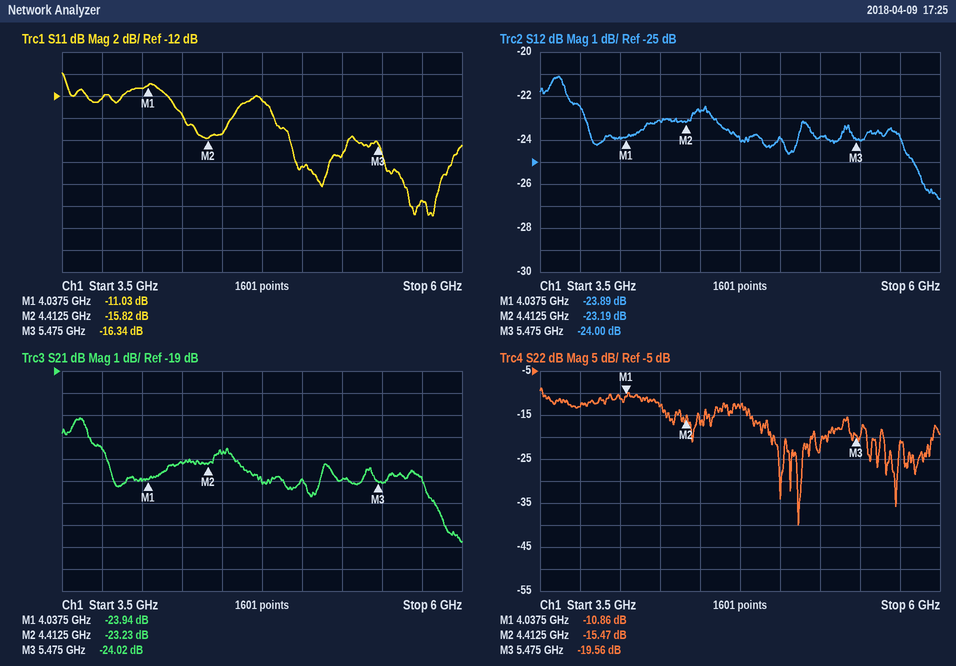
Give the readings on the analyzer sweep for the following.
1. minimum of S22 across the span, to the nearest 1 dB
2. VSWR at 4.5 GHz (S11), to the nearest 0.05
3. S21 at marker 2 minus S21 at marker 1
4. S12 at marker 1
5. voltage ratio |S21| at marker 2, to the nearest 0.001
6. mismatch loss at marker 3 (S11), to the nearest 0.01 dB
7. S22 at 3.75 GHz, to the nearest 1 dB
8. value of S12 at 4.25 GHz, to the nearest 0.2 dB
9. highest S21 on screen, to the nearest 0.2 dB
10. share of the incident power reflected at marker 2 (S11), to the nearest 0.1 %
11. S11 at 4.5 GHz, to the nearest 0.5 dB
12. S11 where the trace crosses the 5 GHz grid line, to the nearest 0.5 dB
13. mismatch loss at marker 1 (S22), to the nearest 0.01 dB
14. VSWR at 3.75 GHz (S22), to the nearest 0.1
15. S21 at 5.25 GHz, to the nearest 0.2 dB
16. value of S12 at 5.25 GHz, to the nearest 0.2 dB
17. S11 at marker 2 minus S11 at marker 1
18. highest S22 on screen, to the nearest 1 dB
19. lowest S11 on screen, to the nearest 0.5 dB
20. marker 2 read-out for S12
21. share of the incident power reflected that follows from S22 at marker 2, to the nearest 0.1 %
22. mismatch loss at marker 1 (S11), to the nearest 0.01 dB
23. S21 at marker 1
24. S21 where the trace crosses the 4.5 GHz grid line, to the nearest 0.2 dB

-40 dB
1.40
0.71 dB
-23.89 dB
0.069
0.10 dB
-13 dB
-23.2 dB
-21.2 dB
2.6 %
-15.5 dB
-18.5 dB
0.37 dB
1.6
-24.0 dB
-23.8 dB
-4.79 dB
-9 dB
-23.0 dB
-23.19 dB
2.8 %
0.36 dB
-23.94 dB
-22.8 dB
